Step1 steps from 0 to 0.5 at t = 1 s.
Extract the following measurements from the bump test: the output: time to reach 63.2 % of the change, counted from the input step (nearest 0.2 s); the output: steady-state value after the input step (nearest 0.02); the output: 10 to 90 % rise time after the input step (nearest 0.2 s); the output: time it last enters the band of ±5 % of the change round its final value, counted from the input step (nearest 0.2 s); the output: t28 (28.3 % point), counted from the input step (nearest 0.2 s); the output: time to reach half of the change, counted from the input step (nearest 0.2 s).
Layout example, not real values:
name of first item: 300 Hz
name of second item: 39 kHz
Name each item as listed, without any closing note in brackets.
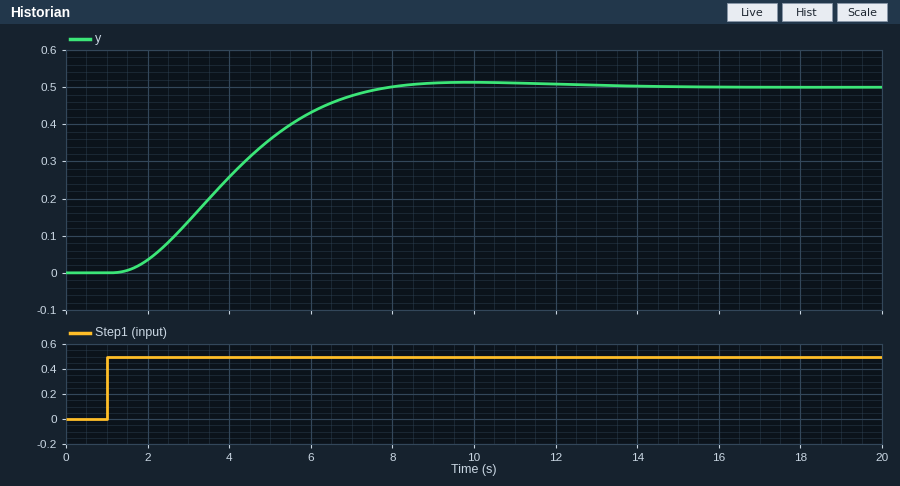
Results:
the output: time to reach 63.2 % of the change, counted from the input step: 3.6 s
the output: steady-state value after the input step: 0.50
the output: 10 to 90 % rise time after the input step: 4.2 s
the output: time it last enters the band of ±5 % of the change round its final value, counted from the input step: 6.0 s
the output: t28 (28.3 % point), counted from the input step: 2.0 s
the output: time to reach half of the change, counted from the input step: 3.0 s
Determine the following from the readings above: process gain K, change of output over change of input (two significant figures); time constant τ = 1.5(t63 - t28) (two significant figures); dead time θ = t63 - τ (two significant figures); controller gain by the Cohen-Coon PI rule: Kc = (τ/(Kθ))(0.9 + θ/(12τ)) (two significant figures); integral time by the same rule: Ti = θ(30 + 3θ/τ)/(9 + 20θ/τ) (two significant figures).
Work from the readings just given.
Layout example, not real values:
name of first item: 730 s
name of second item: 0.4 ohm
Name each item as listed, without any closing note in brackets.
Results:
process gain K, change of output over change of input: 1.0
time constant τ = 1.5(t63 - t28): 2.4 s
dead time θ = t63 - τ: 1.2 s
controller gain by the Cohen-Coon PI rule: Kc = (τ/(Kθ))(0.9 + θ/(12τ)): 1.9
integral time by the same rule: Ti = θ(30 + 3θ/τ)/(9 + 20θ/τ): 2.0 s
